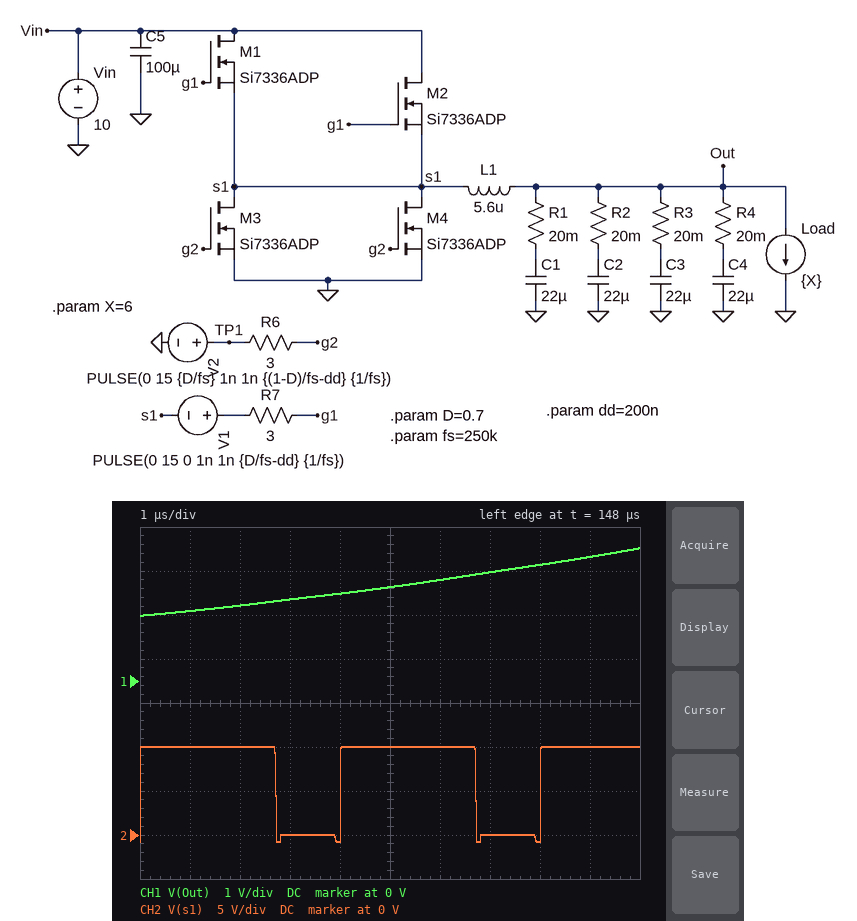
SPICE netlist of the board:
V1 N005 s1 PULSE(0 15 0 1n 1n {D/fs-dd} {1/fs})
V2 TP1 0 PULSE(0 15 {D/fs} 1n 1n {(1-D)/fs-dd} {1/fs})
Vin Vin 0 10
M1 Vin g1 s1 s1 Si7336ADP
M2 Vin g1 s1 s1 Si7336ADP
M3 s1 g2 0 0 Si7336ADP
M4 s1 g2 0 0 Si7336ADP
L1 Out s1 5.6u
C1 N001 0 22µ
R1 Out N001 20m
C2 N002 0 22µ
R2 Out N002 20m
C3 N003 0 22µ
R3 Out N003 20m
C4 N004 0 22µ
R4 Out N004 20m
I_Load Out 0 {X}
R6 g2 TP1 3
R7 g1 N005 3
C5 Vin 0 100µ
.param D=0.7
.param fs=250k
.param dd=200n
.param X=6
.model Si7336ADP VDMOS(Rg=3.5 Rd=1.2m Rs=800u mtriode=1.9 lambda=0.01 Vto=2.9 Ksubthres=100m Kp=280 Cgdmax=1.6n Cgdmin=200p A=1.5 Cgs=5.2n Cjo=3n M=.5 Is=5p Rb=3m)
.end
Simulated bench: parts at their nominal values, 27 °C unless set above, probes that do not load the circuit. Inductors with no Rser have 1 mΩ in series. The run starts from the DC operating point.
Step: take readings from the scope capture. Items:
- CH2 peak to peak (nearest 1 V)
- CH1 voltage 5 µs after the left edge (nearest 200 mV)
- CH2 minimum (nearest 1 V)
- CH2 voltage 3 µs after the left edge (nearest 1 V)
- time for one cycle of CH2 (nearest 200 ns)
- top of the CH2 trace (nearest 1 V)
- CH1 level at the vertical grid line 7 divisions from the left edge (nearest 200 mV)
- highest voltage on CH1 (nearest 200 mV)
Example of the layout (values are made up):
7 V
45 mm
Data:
11 V
2.2 V
-1 V
0 V
4.0 µs
10 V
2.4 V
3.0 V
